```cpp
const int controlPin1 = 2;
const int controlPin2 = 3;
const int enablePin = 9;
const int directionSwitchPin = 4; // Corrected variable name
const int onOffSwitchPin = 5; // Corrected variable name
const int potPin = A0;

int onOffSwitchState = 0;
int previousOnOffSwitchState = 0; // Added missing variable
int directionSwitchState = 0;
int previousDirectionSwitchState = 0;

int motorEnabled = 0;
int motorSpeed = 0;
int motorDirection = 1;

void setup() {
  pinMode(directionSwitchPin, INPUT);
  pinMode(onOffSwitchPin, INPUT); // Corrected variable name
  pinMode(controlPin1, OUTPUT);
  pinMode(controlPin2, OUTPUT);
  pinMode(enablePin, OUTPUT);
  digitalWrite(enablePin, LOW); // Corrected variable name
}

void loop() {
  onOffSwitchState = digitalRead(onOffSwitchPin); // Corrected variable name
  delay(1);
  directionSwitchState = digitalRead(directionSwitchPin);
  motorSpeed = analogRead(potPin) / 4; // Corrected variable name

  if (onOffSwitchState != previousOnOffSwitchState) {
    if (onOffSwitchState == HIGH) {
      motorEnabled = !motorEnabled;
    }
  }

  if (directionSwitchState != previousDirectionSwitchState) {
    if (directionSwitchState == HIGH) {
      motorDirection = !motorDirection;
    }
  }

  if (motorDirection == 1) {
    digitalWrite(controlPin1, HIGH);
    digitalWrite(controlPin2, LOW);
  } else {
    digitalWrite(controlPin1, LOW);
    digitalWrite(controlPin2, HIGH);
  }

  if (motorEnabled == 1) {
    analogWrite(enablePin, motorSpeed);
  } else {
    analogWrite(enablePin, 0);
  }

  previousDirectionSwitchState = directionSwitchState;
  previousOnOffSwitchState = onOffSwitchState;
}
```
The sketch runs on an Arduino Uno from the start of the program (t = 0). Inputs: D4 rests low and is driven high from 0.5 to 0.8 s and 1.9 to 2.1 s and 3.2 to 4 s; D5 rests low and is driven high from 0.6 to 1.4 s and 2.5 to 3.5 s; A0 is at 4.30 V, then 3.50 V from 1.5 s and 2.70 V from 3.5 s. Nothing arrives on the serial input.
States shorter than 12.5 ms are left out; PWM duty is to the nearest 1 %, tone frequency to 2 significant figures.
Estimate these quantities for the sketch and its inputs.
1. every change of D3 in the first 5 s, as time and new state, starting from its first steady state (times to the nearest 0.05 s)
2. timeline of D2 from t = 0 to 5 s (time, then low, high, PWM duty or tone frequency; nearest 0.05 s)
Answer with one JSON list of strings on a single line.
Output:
["0 s low; 0.5 s high; 1.9 s low; 3.2 s high", "0 s high; 0.5 s low; 1.9 s high; 3.2 s low"]
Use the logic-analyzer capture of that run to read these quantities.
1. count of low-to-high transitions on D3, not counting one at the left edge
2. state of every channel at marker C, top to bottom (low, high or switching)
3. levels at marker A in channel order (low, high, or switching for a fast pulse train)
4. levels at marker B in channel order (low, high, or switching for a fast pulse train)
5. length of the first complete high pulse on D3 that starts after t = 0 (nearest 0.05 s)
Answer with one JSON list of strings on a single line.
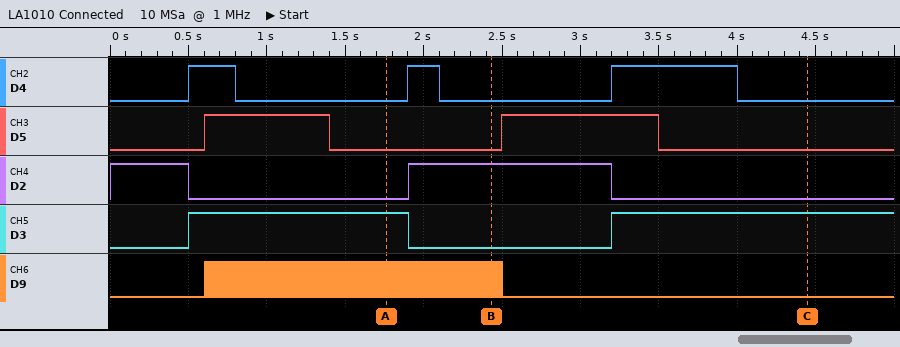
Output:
["2", "D4 low, D5 low, D2 low, D3 high, D9 low", "D4 low, D5 low, D2 low, D3 high, D9 switching", "D4 low, D5 low, D2 high, D3 low, D9 switching", "1.40 s"]
